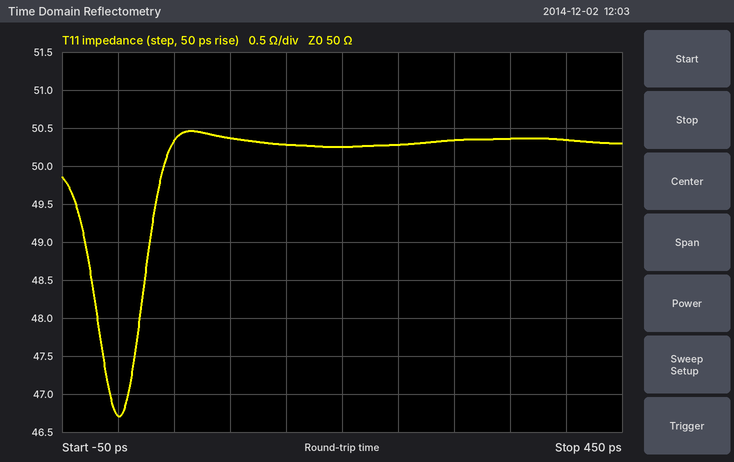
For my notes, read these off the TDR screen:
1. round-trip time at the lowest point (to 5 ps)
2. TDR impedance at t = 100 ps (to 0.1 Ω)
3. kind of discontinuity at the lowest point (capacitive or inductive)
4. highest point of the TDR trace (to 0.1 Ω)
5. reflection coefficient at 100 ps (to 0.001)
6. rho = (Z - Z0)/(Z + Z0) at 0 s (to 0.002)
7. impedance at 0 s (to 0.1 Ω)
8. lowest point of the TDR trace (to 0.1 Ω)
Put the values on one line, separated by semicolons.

0 ps; 50.4 Ω; capacitive; 50.5 Ω; +0.004; -0.034; 46.7 Ω; 46.7 Ω
